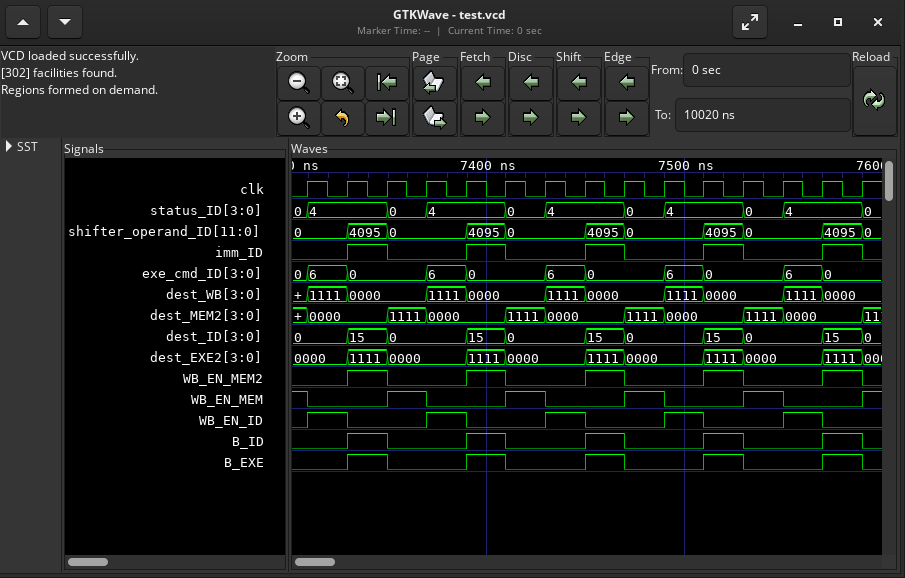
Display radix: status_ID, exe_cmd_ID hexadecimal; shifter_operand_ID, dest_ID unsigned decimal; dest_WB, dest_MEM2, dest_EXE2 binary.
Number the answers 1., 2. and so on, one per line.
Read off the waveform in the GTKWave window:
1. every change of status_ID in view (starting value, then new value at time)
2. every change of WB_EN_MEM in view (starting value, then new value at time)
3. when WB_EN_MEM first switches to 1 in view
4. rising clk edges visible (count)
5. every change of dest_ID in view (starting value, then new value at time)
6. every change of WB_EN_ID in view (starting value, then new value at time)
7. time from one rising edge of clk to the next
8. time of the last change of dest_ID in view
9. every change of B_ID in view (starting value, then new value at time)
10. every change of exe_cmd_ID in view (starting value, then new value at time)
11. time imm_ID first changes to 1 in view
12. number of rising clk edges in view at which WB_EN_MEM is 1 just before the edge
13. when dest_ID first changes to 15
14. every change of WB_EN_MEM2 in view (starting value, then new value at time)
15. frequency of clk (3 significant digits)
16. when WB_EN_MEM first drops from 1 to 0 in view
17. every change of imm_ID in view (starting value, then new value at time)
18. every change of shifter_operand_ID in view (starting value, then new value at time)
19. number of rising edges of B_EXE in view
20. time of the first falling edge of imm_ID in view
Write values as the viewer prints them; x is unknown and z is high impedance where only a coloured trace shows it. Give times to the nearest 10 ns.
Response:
1. 0, 4 at 7310 ns, 0 at 7350 ns, 4 at 7370 ns, 0 at 7410 ns, 4 at 7430 ns, 0 at 7470 ns, 4 at 7490 ns, 0 at 7530 ns, 4 at 7550 ns, 0 at 7590 ns
2. 1, 0 at 7310 ns, 1 at 7350 ns, 0 at 7370 ns, 1 at 7410 ns, 0 at 7430 ns, 1 at 7470 ns, 0 at 7490 ns, 1 at 7530 ns, 0 at 7550 ns, 1 at 7590 ns
3. 7350 ns
4. 15
5. 0, 15 at 7330 ns, 0 at 7350 ns, 15 at 7390 ns, 0 at 7410 ns, 15 at 7450 ns, 0 at 7470 ns, 15 at 7510 ns, 0 at 7530 ns, 15 at 7570 ns, 0 at 7590 ns
6. 0, 1 at 7310 ns, 0 at 7330 ns, 1 at 7370 ns, 0 at 7390 ns, 1 at 7430 ns, 0 at 7450 ns, 1 at 7490 ns, 0 at 7510 ns, 1 at 7550 ns, 0 at 7570 ns
7. 20 ns
8. 7590 ns
9. 0, 1 at 7330 ns, 0 at 7350 ns, 1 at 7390 ns, 0 at 7410 ns, 1 at 7450 ns, 0 at 7470 ns, 1 at 7510 ns, 0 at 7530 ns, 1 at 7570 ns, 0 at 7590 ns
10. 0, 6 at 7310 ns, 0 at 7330 ns, 6 at 7370 ns, 0 at 7390 ns, 6 at 7430 ns, 0 at 7450 ns, 6 at 7490 ns, 0 at 7510 ns, 6 at 7550 ns, 0 at 7570 ns
11. 7330 ns
12. 5
13. 7330 ns
14. 0, 1 at 7330 ns, 0 at 7350 ns, 1 at 7390 ns, 0 at 7410 ns, 1 at 7450 ns, 0 at 7470 ns, 1 at 7510 ns, 0 at 7530 ns, 1 at 7570 ns, 0 at 7590 ns
15. 50.0 MHz
16. 7310 ns
17. 0, 1 at 7330 ns, 0 at 7350 ns, 1 at 7390 ns, 0 at 7410 ns, 1 at 7450 ns, 0 at 7470 ns, 1 at 7510 ns, 0 at 7530 ns, 1 at 7570 ns, 0 at 7590 ns
18. 0, 4095 at 7330 ns, 0 at 7350 ns, 4095 at 7390 ns, 0 at 7410 ns, 4095 at 7450 ns, 0 at 7470 ns, 4095 at 7510 ns, 0 at 7530 ns, 4095 at 7570 ns, 0 at 7590 ns
19. 5
20. 7350 ns
